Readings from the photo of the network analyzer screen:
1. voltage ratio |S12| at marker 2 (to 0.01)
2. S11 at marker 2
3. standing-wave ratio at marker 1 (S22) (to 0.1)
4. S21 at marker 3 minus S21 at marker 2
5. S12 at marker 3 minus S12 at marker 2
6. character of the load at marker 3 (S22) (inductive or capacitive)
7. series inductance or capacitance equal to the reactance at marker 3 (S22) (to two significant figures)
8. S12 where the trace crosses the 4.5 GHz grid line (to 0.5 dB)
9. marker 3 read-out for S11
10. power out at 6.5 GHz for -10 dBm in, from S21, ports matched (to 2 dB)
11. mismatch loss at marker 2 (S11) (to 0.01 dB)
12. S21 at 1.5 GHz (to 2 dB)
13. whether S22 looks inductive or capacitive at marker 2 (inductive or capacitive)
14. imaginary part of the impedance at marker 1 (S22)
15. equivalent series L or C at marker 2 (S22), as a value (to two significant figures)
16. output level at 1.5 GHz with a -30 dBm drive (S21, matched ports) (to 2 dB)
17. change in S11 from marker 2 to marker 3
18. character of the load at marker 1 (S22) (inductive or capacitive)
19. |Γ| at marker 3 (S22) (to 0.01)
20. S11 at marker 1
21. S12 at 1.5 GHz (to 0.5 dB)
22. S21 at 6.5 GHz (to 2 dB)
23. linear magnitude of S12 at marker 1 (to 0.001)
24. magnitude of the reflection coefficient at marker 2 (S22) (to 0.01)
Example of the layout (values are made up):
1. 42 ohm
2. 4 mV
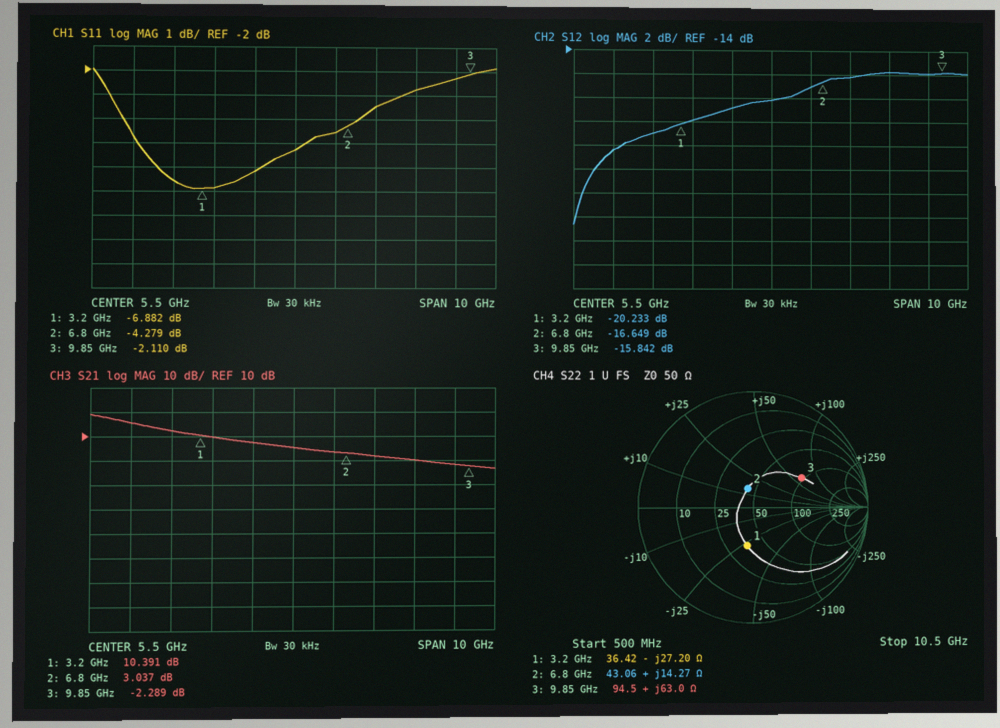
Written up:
1. 0.15
2. -4.279 dB
3. 2.0
4. -5.326 dB
5. 0.807 dB
6. inductive
7. 1.0 nH
8. -19.0 dB
9. -2.110 dB
10. -6 dBm
11. 2.03 dB
12. 16 dB
13. inductive
14. -27.20 Ω
15. 330 pH
16. -14 dBm
17. 2.169 dB
18. capacitive
19. 0.49
20. -6.882 dB
21. -22.5 dB
22. 4 dB
23. 0.097
24. 0.17
